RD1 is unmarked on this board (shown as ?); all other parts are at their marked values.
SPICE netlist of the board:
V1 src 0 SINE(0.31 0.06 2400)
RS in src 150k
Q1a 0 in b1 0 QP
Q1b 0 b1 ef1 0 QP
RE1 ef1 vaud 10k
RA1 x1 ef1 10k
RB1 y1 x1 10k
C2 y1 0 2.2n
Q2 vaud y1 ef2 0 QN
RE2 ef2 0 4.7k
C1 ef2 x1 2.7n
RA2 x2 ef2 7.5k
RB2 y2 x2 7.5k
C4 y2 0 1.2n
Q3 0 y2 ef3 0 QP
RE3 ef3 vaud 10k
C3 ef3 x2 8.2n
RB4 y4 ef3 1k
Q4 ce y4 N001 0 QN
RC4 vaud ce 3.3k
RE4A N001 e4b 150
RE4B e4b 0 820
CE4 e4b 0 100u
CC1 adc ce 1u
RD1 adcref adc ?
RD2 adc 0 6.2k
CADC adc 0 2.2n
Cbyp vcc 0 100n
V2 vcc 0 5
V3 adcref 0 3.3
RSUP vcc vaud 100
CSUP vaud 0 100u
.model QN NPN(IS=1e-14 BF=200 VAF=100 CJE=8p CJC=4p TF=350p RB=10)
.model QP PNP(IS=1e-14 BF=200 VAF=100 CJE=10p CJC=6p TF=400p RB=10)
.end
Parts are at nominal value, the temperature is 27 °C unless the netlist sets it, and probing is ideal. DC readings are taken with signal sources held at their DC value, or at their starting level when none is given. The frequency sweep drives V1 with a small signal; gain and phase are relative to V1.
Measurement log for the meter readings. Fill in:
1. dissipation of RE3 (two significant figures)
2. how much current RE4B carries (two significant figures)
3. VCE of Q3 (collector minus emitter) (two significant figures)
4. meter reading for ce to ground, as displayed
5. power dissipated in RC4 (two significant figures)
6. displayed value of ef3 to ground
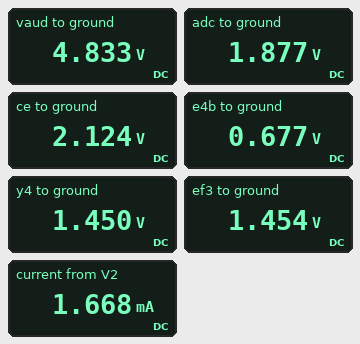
1.1 mW
830 µA
-1.5 V
2.124 V
2.2 mW
1.454 V
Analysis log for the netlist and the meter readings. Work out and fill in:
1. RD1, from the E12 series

4.7 kΩ
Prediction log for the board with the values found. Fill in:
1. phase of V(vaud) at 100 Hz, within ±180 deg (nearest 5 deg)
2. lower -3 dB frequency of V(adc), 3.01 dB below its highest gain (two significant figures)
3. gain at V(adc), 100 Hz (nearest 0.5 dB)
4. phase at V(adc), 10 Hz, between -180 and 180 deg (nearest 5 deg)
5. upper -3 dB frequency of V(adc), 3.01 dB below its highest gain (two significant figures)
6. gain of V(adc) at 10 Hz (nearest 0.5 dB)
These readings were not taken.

85 deg
30 Hz
17.0 dB
-75 deg
6.1 kHz
5.0 dB
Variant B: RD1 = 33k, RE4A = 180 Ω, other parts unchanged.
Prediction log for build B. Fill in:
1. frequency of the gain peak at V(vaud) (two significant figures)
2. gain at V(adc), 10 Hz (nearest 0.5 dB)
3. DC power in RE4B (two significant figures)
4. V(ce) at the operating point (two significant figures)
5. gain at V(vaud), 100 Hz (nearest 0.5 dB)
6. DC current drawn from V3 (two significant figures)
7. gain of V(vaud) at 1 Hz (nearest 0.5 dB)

10 Hz
9.5 dB
530 µW
2.2 V
-27.5 dB
84 µA
-20.5 dB
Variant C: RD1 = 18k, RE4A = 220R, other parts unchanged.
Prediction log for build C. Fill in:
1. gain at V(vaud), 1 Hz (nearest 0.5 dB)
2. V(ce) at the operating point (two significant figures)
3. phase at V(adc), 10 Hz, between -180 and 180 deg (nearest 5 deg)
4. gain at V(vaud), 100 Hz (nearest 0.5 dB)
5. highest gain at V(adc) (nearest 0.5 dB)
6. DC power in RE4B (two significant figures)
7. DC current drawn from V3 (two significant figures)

-20.5 dB
2.3 V
-90 deg
-29.5 dB
16.5 dB
490 µW
140 µA
